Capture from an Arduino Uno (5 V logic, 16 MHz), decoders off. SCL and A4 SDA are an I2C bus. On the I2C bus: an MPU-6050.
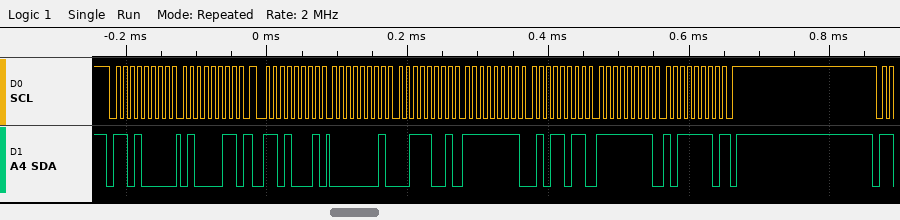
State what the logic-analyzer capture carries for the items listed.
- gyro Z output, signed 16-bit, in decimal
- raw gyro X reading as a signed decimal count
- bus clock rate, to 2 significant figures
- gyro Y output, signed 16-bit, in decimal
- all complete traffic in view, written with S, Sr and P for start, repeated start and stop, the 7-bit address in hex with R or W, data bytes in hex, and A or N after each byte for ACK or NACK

-66
313
100 kHz
-165
S 68W A 43 A Sr 68R A 01 A 39 A FF A 5B A FF A BE N P
